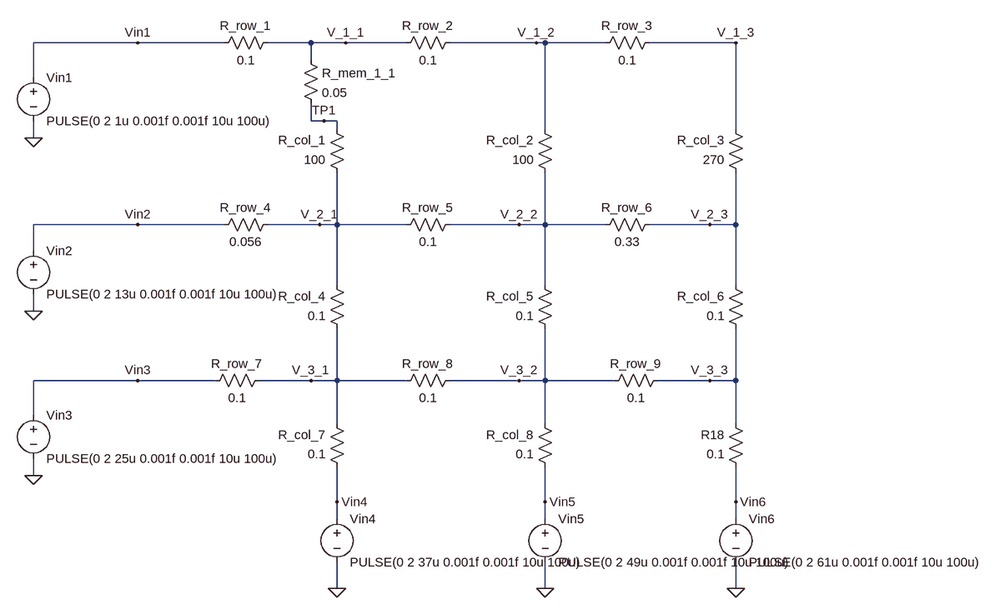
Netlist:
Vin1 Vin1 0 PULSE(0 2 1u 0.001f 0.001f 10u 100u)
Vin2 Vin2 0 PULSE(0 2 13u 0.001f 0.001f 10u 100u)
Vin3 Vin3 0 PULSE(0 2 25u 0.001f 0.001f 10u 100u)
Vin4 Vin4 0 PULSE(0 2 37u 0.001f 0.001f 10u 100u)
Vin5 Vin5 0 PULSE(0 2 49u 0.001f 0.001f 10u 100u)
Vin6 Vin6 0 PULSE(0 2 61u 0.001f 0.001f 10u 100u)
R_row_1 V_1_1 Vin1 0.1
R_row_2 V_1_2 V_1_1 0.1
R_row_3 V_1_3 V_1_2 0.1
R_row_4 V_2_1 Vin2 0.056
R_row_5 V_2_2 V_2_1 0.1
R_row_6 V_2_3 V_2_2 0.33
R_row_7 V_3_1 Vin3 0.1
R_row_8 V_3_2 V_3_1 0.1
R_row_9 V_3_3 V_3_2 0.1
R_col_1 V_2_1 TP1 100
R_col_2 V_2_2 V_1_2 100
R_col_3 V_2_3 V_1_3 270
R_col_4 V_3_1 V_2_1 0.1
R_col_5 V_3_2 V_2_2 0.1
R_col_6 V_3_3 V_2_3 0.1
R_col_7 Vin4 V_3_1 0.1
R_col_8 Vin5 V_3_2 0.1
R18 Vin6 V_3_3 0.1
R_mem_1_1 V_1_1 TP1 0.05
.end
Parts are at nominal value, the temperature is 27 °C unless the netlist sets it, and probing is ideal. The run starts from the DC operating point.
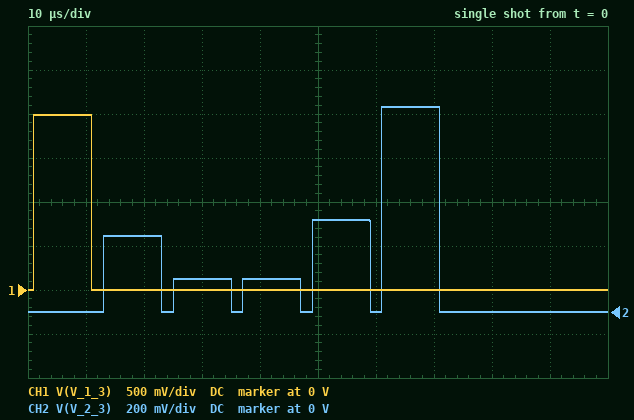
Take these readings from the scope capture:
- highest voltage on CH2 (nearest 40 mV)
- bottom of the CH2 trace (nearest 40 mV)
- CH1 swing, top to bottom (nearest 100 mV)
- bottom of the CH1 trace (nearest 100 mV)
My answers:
920 mV
0 V
2.0 V
0 V
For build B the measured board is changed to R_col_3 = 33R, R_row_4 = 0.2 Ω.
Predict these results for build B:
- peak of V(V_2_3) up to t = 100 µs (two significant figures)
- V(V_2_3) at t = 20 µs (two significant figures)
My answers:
960 mV
170 mV
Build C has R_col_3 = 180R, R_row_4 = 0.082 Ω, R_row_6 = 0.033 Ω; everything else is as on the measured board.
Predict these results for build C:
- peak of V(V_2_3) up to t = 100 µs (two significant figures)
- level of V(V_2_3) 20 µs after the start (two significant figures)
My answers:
630 mV
470 mV
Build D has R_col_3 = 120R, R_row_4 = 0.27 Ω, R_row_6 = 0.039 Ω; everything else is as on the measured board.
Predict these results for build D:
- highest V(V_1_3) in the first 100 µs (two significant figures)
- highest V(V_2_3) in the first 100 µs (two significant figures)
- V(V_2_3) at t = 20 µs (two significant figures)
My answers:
2.0 V
700 mV
220 mV
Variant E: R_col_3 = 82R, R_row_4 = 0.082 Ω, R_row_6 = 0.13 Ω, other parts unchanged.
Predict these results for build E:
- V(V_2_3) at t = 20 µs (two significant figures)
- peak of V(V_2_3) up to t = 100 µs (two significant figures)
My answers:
380 mV
790 mV
